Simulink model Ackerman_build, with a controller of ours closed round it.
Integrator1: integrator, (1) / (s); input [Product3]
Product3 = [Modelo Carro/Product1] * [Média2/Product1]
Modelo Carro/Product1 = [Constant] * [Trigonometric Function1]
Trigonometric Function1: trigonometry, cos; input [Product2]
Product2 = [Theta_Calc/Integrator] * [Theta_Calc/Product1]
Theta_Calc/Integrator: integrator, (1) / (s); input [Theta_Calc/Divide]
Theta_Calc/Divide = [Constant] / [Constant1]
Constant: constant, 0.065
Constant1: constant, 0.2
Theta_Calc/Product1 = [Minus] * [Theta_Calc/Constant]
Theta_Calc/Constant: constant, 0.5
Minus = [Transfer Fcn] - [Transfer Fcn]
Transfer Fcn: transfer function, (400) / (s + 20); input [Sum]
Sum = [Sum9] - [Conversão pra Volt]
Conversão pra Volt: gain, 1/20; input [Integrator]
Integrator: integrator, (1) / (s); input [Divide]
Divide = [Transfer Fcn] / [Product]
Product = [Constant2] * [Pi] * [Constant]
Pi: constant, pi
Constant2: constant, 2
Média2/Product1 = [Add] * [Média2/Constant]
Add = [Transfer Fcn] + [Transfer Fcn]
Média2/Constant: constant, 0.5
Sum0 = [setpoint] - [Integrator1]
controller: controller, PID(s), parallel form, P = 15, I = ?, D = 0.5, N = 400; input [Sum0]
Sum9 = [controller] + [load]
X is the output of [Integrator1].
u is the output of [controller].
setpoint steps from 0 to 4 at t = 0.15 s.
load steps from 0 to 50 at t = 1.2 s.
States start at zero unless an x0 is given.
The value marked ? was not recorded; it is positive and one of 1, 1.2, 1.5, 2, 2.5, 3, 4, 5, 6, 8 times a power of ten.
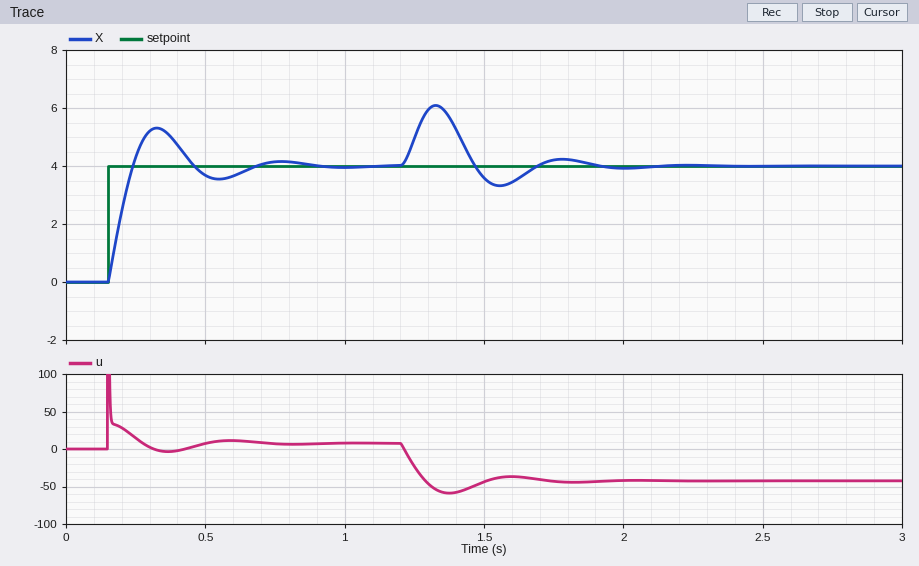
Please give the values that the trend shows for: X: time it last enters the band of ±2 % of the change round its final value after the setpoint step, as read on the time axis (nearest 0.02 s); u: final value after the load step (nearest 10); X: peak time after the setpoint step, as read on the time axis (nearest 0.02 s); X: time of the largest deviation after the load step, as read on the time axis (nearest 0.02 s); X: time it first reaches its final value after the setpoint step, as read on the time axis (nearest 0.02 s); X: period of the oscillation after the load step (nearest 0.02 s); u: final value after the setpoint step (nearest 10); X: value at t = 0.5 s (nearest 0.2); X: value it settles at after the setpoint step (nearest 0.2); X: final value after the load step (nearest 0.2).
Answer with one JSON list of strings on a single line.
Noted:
["0.86 s", "-40", "0.32 s", "1.32 s", "0.24 s", "0.46 s", "10", "3.6", "4.0", "4.0"]
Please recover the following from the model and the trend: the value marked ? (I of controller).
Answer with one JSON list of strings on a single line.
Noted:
["200"]
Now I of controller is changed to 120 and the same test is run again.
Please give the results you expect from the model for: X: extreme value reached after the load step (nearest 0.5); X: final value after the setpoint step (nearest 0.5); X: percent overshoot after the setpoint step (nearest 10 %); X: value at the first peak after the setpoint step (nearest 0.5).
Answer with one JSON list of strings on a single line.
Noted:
["6.5", "4.0", "20 %", "5.0"]
